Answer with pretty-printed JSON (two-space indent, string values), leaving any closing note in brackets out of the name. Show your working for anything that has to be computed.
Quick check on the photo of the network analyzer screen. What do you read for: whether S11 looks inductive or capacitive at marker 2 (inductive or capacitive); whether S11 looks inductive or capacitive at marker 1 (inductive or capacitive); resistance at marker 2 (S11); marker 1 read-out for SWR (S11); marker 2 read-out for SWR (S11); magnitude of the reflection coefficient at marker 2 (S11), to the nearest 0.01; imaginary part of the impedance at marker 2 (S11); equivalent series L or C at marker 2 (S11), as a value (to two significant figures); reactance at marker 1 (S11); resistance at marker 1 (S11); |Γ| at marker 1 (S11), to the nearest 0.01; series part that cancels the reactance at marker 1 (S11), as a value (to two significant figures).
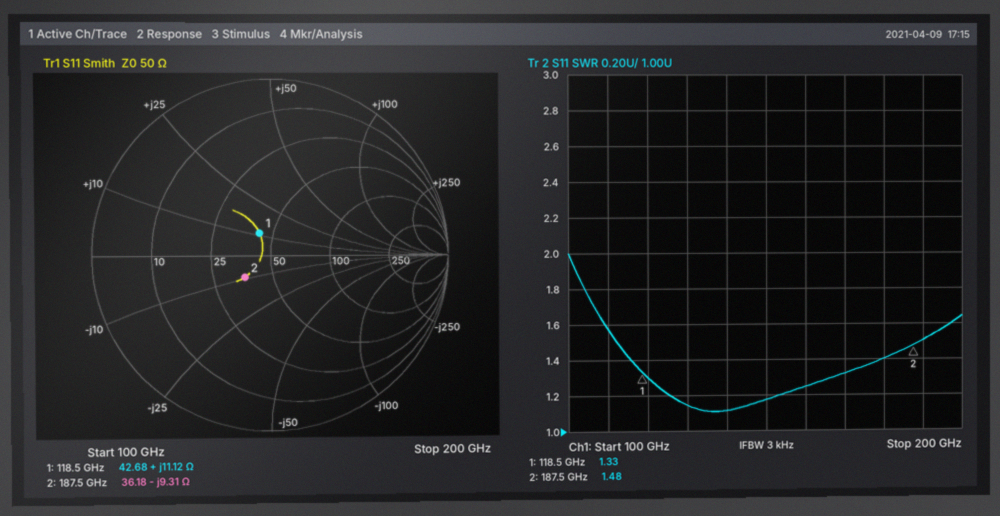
{
  "whether S11 looks inductive or capacitive at marker 2": "capacitive",
  "whether S11 looks inductive or capacitive at marker 1": "inductive",
  "resistance at marker 2": "36.18 Ω",
  "marker 1 read-out for SWR": "1.33",
  "marker 2 read-out for SWR": "1.48",
  "magnitude of the reflection coefficient at marker 2 (S11), to the nearest 0.01": "0.19",
  "imaginary part of the impedance at marker 2": "-9.31 Ω",
  "equivalent series L or C at marker 2 (S11), as a value": "C = 1/(2π × 187.5 GHz × 9.31 Ω) ≈ 91 fF",
  "reactance at marker 1": "+11.12 Ω",
  "resistance at marker 1": "42.68 Ω",
  "|Γ| at marker 1 (S11), to the nearest 0.01": "0.14",
  "series part that cancels the reactance at marker 1 (S11), as a value": "C = 1/(2π × 118.5 GHz × 11.12 Ω) ≈ 121 fF, so 120 fF to two significant figures"
}
